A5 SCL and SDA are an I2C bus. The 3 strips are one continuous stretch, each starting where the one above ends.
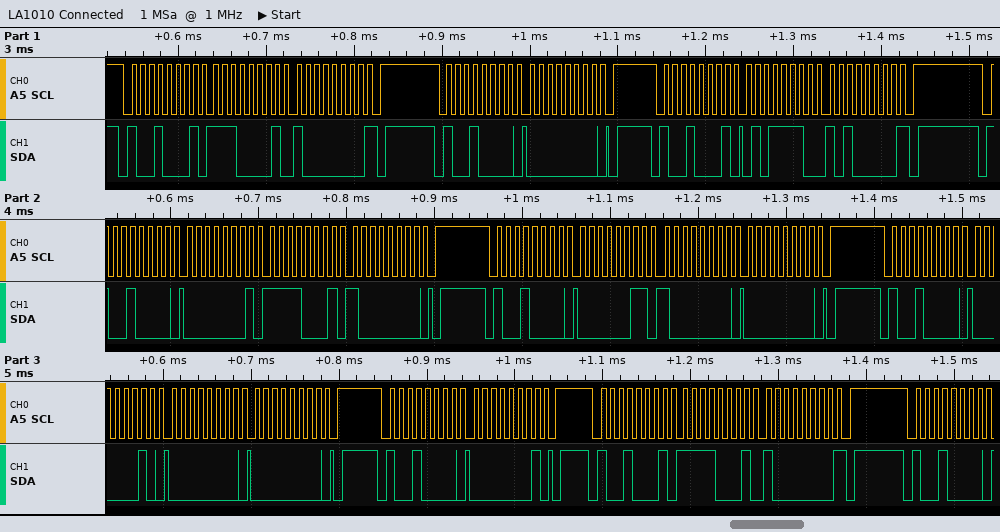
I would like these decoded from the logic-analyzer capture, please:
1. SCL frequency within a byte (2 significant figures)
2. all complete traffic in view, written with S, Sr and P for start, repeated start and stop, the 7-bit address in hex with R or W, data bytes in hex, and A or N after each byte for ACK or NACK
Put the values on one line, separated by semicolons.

100 kHz; S 48R A E1 A 80 N P S 48W A 00 A P S 48R A 5E A A0 N P S 48W A 01 A F1 A 80 A P S 48W A 03 A 80 A 00 A P S 48W A 02 A 00 A 00 A P S 48W A 01 A P S 48R A F1 A 80 N P S 48W A
